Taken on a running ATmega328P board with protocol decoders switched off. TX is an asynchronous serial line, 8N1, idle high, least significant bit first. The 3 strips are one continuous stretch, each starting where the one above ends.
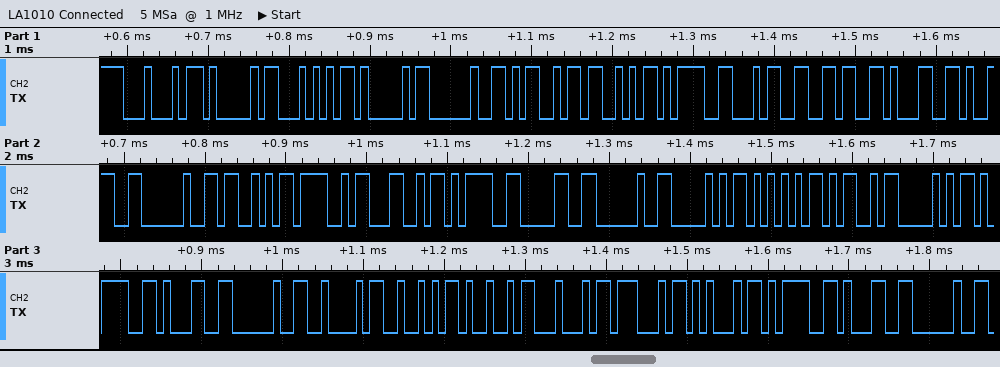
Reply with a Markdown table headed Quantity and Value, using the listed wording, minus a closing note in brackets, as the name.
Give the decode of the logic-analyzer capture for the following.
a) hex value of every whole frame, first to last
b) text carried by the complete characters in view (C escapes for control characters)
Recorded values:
| Quantity | Value |
|---|---|
| hex value of every whole frame, first to last | 44 41 54 41 20 4D 53 3D 34 36 31 39 20 53 4F 4C 3D 30 20 50 55 4D 50 3D 31 20 42 52 49 44 47 45 3D 31 20 |
| text carried by the complete characters in view | "DATA MS=4619 SOL=0 PUMP=1 BRIDGE=1 " |
